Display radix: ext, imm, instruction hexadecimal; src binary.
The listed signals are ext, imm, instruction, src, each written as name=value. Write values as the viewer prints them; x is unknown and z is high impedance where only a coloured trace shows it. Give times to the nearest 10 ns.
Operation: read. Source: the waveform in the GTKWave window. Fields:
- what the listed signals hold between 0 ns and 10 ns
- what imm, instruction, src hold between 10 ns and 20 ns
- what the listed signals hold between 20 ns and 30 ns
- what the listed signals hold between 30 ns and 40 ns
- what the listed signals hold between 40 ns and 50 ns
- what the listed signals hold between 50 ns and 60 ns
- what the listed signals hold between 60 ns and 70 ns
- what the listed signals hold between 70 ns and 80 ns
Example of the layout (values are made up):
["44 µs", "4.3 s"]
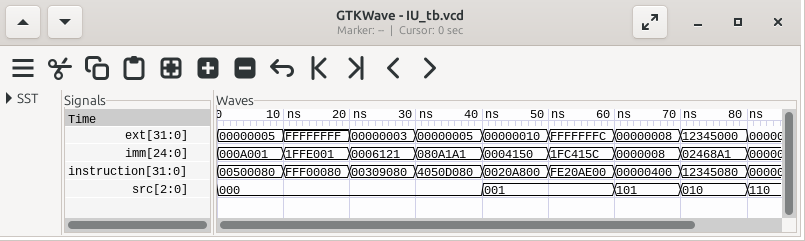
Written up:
["ext=00000005, imm=000A001, instruction=00500080, src=000", "imm=1FFE001, instruction=FFF00080, src=000", "ext=00000003, imm=0006121, instruction=00309080, src=000", "ext=00000005, imm=080A1A1, instruction=4050D080, src=000", "ext=00000010, imm=0004150, instruction=0020A800, src=001", "ext=FFFFFFFC, imm=1FC415C, instruction=FE20AE00, src=001", "ext=00000008, imm=0000008, instruction=00000400, src=101", "ext=12345000, imm=02468A1, instruction=12345080, src=010"]
